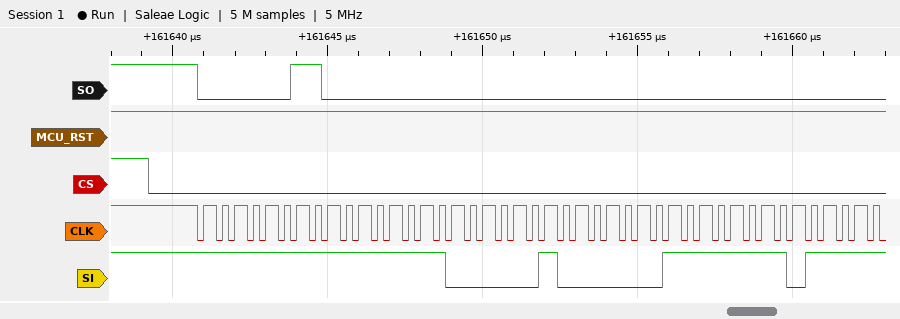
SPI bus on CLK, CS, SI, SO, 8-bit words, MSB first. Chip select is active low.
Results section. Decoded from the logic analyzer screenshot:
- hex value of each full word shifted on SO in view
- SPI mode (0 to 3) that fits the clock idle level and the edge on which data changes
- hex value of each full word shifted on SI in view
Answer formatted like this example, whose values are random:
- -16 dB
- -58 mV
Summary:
- 03, 00, 00, 00, 00
- 3
- FF, FF, 02, 03, FD
